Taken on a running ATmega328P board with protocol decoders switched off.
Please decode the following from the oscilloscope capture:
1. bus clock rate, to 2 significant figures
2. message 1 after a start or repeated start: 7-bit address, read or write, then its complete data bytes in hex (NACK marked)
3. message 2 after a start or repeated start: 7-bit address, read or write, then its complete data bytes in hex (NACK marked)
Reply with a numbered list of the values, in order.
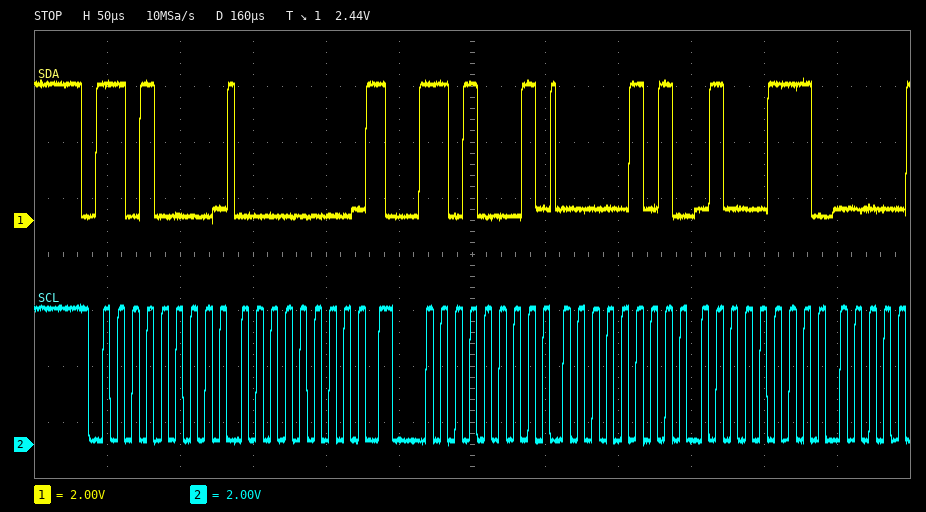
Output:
1. 100 kHz
2. 0x68 write: 00
3. 0x68 read: 05 47
